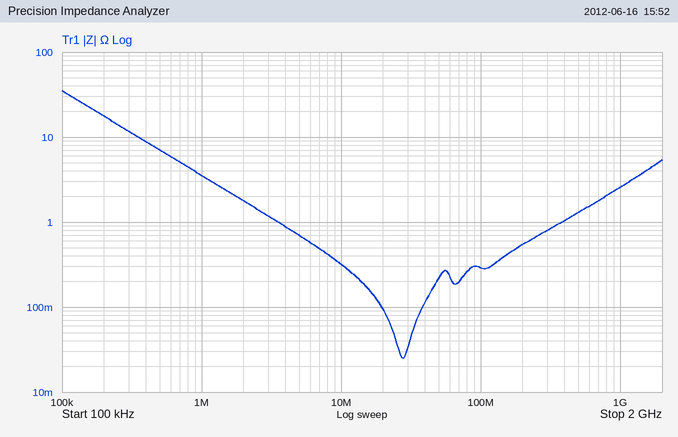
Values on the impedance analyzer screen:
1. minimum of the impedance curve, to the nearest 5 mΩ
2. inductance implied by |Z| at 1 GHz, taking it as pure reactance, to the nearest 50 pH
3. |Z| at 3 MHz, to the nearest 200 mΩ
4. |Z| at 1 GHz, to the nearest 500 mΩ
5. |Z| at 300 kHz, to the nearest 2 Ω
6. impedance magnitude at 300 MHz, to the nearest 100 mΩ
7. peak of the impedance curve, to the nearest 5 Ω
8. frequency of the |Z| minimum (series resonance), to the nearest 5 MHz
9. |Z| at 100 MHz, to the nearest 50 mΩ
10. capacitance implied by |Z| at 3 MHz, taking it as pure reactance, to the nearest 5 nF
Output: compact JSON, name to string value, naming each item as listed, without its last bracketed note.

{"minimum of the impedance curve, to the nearest 5 mΩ": "25 mΩ", "inductance implied by |Z| at 1 GHz, taking it as pure reactance, to the nearest 50 pH": "400 pH", "|Z| at 3 MHz, to the nearest 200 mΩ": "1.2 Ω", "|Z| at 1 GHz, to the nearest 500 mΩ": "2.5 Ω", "|Z| at 300 kHz, to the nearest 2 Ω": "12 Ω", "impedance magnitude at 300 MHz, to the nearest 100 mΩ": "800 mΩ", "peak of the impedance curve, to the nearest 5 Ω": "35 Ω", "frequency of the |Z| minimum (series resonance), to the nearest 5 MHz": "30 MHz", "|Z| at 100 MHz, to the nearest 50 mΩ": "300 mΩ", "capacitance implied by |Z| at 3 MHz, taking it as pure reactance, to the nearest 5 nF": "45 nF"}
